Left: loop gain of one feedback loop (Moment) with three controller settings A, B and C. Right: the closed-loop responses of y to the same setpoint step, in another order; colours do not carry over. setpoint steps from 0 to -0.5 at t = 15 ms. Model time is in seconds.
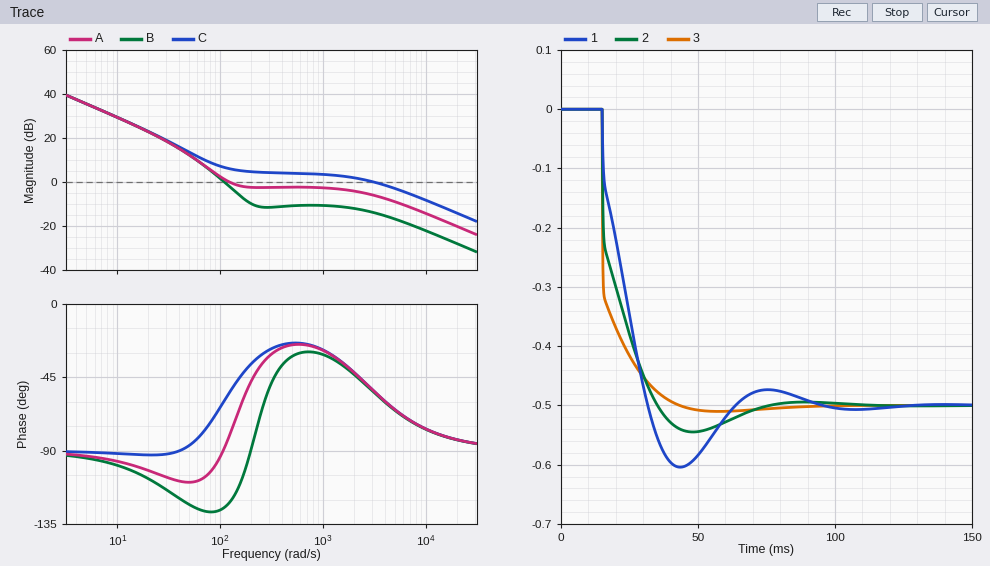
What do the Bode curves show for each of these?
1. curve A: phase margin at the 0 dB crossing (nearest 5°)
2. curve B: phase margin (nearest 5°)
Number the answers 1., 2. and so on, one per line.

1. 100°
2. 55°
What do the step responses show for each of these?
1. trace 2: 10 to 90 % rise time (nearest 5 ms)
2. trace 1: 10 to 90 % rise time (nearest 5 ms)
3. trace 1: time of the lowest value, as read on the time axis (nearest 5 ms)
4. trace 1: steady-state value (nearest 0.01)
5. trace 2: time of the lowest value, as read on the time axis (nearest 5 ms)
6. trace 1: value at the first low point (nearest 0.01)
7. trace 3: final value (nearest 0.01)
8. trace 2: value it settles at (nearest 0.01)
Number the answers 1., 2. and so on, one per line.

1. 15 ms
2. 15 ms
3. 45 ms
4. -0.50
5. 50 ms
6. -0.60
7. -0.50
8. -0.50
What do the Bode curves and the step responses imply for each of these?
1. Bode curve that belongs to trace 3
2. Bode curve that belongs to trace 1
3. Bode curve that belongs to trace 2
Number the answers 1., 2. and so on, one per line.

1. C
2. B
3. A
